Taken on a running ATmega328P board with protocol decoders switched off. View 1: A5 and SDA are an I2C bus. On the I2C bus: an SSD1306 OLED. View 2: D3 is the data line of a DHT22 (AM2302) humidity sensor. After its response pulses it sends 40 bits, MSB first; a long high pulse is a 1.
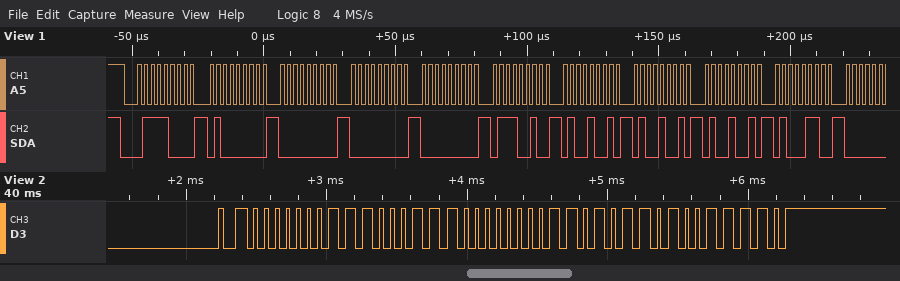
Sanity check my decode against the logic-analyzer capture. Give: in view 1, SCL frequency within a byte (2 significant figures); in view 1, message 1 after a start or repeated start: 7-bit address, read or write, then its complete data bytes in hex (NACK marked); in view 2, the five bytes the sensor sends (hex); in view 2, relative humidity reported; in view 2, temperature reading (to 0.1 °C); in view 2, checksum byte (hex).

400 kHz
0x3C write: 40 00 00 00 72 49 49 49 46
01 C7 00 D6 9E
45.5 %
21.4 °C
0x9E
